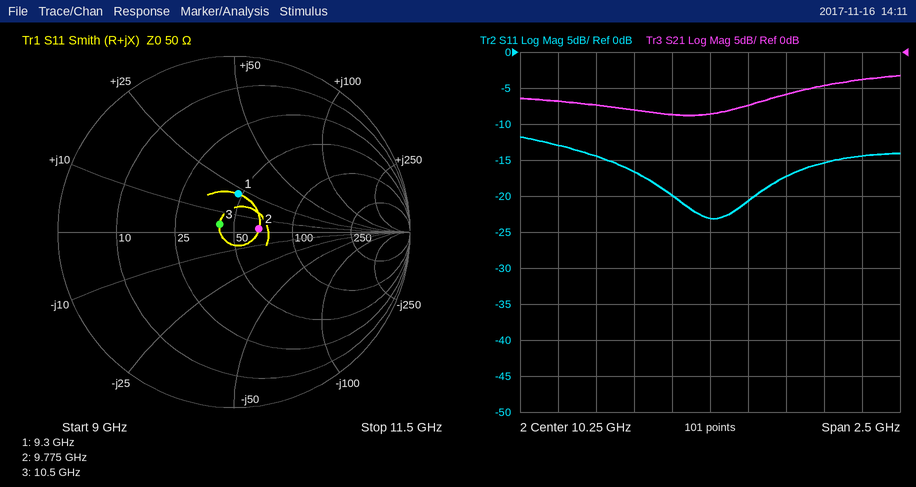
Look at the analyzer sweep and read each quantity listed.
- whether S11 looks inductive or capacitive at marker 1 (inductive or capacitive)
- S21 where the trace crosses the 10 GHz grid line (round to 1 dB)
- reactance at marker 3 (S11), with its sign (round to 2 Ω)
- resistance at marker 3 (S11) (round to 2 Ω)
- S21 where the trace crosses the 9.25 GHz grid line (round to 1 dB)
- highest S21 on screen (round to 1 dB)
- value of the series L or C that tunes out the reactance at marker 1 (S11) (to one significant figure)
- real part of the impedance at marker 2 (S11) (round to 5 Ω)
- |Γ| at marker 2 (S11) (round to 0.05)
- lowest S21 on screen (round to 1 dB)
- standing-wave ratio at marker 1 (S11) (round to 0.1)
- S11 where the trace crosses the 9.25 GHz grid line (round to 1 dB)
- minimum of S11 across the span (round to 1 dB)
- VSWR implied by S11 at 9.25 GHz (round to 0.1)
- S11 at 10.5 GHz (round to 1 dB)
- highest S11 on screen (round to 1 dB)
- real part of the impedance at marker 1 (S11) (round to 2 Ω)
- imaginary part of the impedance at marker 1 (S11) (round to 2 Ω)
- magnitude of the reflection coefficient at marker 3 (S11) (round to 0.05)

inductive
-9 dB
+4 Ω
42 Ω
-7 dB
-3 dB
800 fF
65 Ω
0.15
-9 dB
1.6
-13 dB
-23 dB
1.6
-21 dB
-12 dB
48 Ω
+22 Ω
0.10
